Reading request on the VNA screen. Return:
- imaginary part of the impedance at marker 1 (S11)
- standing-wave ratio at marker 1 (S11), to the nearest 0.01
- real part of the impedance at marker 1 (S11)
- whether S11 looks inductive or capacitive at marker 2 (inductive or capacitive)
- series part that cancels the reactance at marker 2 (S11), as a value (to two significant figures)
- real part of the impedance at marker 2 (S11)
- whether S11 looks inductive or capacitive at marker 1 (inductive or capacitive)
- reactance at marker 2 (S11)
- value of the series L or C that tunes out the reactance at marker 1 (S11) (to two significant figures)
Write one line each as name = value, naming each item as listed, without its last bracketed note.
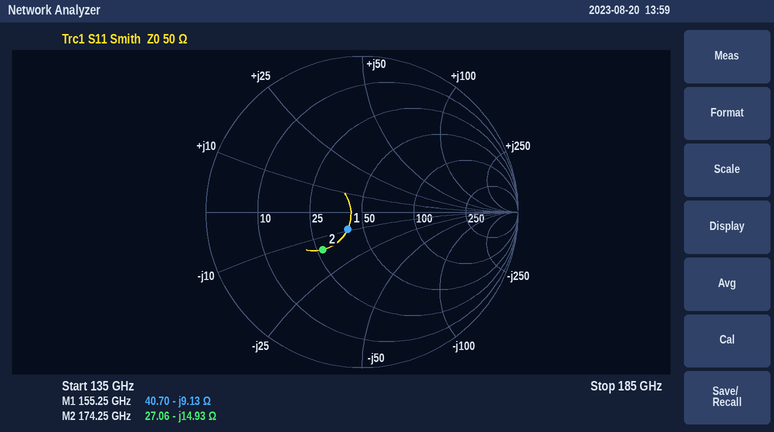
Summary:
imaginary part of the impedance at marker 1 = -9.13 Ω
standing-wave ratio at marker 1 (S11), to the nearest 0.01 = 1.33
real part of the impedance at marker 1 = 40.70 Ω
whether S11 looks inductive or capacitive at marker 2 = capacitive
series part that cancels the reactance at marker 2 (S11), as a value = 14 pH
real part of the impedance at marker 2 = 27.06 Ω
whether S11 looks inductive or capacitive at marker 1 = capacitive
reactance at marker 2 = -14.93 Ω
value of the series L or C that tunes out the reactance at marker 1 (S11) = 9.4 pH
